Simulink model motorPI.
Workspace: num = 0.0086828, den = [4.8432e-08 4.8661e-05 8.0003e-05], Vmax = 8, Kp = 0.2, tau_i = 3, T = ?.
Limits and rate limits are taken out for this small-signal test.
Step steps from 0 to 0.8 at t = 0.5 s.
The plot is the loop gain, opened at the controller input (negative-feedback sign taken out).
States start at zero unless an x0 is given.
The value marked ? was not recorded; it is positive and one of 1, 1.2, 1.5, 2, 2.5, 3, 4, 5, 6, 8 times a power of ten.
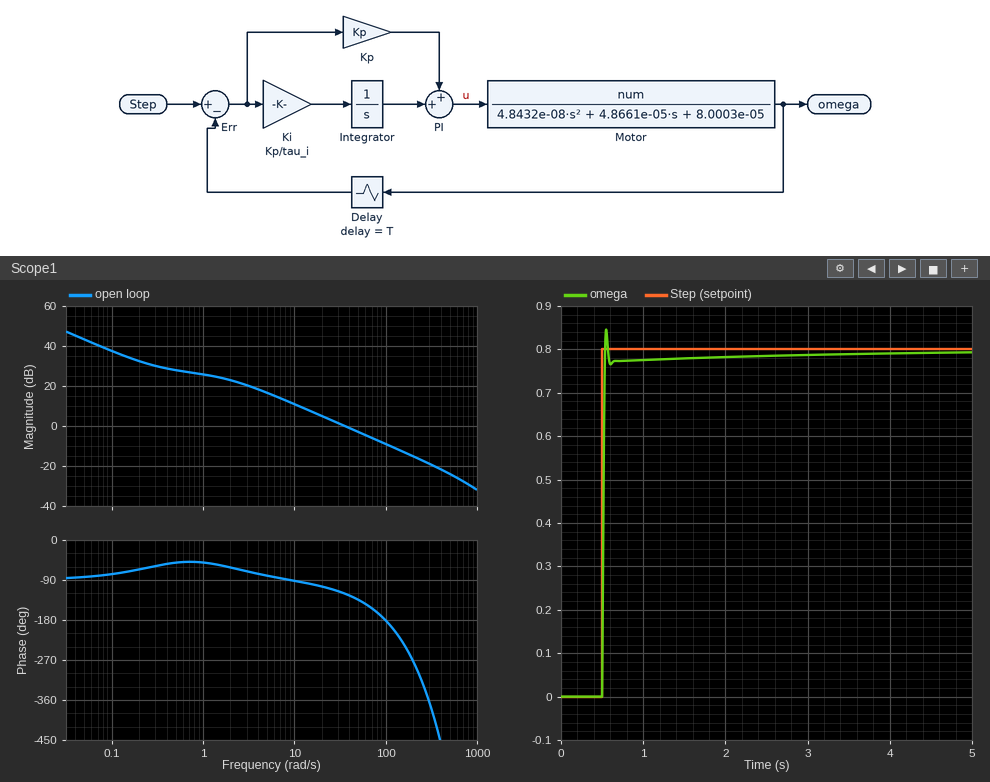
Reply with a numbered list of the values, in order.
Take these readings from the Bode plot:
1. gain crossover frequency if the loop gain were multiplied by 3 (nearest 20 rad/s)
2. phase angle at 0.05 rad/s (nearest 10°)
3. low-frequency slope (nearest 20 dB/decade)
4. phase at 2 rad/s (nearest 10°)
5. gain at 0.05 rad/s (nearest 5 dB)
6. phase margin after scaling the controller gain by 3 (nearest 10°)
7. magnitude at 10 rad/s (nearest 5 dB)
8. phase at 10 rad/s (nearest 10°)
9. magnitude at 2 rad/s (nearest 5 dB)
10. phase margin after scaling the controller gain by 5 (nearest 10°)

1. 100 rad/s
2. -80°
3. -20 dB/decade
4. -60°
5. 45 dB
6. -10°
7. 10 dB
8. -90°
9. 25 dB
10. -70°
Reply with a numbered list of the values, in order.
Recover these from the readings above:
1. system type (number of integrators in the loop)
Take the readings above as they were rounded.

1. 1
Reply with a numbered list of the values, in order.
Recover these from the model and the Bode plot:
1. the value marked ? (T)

1. 0.015
